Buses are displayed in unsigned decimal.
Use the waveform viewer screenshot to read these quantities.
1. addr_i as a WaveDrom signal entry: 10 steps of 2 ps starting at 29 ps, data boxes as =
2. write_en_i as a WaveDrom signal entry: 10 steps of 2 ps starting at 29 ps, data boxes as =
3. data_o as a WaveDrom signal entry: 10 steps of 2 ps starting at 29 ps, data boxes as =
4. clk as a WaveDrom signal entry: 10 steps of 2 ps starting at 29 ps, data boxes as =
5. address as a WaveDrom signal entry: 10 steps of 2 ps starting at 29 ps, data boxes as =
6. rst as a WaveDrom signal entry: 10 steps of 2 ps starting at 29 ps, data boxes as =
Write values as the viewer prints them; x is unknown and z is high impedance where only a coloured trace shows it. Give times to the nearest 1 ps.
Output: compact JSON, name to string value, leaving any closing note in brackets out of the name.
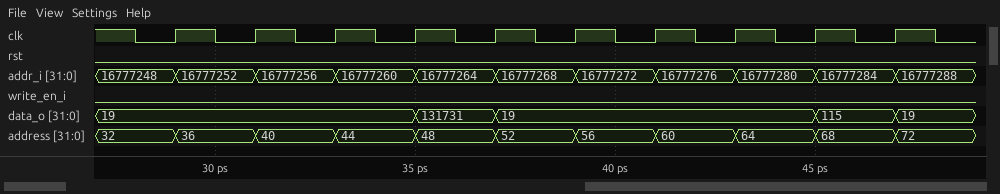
{"addr_i as a WaveDrom signal entry: 10 steps of 2 ps starting at 29 ps, data boxes as =": "{name: 'addr_i', wave: '==========', data: '16777252 16777256 16777260 16777264 16777268 16777272 16777276 16777280 16777284 16777288'}", "write_en_i as a WaveDrom signal entry: 10 steps of 2 ps starting at 29 ps, data boxes as =": "{name: 'write_en_i', wave: '0.........'}", "data_o as a WaveDrom signal entry: 10 steps of 2 ps starting at 29 ps, data boxes as =": "{name: 'data_o', wave: '=..==...==', data: '19 131731 19 115 19'}", "clk as a WaveDrom signal entry: 10 steps of 2 ps starting at 29 ps, data boxes as =": "{name: 'clk', wave: 'p.........'}", "address as a WaveDrom signal entry: 10 steps of 2 ps starting at 29 ps, data boxes as =": "{name: 'address', wave: '==========', data: '36 40 44 48 52 56 60 64 68 72'}", "rst as a WaveDrom signal entry: 10 steps of 2 ps starting at 29 ps, data boxes as =": "{name: 'rst', wave: '0.........'}"}
